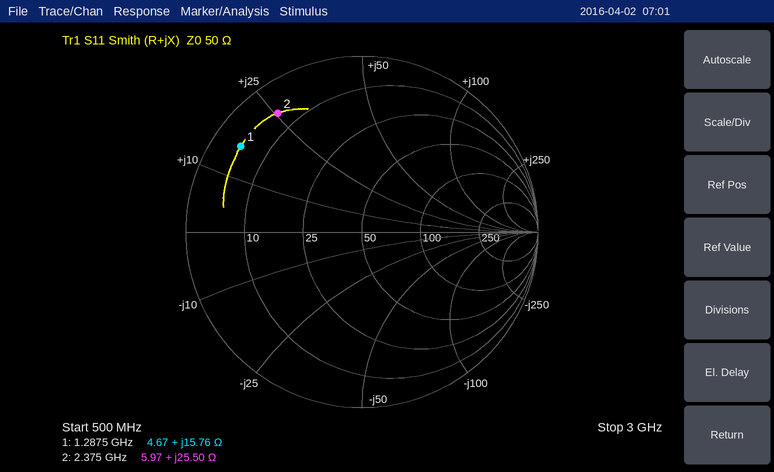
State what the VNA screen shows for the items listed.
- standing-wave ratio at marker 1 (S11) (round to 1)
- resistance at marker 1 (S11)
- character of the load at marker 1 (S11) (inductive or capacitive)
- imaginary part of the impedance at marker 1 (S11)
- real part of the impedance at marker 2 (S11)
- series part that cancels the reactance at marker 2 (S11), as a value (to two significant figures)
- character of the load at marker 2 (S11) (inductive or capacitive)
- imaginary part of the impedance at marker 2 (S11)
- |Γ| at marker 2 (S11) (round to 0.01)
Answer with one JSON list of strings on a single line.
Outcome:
["12", "4.67 Ω", "inductive", "+15.76 Ω", "5.97 Ω", "2.6 pF", "inductive", "+25.50 Ω", "0.83"]
